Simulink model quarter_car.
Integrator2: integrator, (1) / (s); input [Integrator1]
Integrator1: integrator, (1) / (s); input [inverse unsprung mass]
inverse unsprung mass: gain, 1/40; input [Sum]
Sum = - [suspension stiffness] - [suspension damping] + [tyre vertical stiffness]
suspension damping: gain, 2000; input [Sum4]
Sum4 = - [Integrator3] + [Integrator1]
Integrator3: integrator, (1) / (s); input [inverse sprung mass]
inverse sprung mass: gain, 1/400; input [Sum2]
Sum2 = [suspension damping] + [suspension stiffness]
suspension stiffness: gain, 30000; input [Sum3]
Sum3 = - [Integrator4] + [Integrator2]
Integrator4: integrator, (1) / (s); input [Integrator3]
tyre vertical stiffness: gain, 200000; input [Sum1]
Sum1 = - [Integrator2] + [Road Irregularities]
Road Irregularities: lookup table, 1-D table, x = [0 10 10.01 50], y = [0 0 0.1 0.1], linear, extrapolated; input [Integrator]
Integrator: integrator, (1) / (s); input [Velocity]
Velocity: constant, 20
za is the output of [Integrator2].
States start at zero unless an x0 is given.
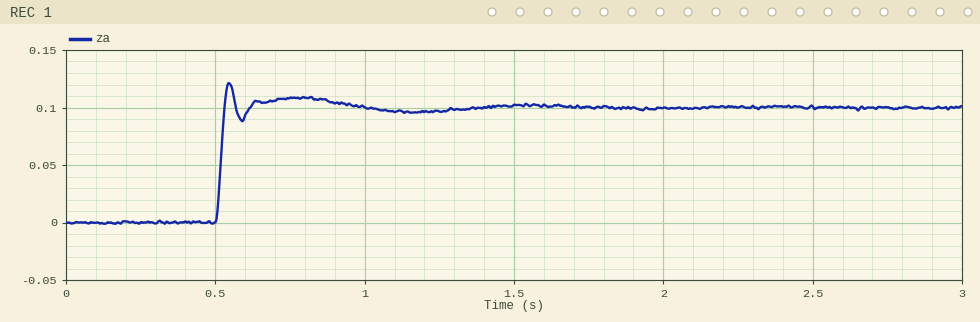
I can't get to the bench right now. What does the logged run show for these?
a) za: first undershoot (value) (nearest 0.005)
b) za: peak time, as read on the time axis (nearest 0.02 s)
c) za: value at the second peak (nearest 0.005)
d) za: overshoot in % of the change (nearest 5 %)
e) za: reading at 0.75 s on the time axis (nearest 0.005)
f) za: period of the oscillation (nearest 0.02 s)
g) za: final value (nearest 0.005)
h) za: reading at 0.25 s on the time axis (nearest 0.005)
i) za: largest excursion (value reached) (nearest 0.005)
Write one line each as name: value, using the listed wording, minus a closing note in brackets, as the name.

za: first undershoot (value): 0.090
za: peak time, as read on the time axis: 0.54 s
za: value at the second peak: 0.110
za: overshoot in % of the change: 20 %
za: reading at 0.75 s on the time axis: 0.110
za: period of the oscillation: 0.24 s
za: final value: 0.100
za: reading at 0.25 s on the time axis: 0.000
za: largest excursion (value reached): 0.120
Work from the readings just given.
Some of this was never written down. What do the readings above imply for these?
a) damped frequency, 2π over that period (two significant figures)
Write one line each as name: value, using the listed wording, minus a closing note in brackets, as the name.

damped frequency, 2π over that period: 26 rad/s
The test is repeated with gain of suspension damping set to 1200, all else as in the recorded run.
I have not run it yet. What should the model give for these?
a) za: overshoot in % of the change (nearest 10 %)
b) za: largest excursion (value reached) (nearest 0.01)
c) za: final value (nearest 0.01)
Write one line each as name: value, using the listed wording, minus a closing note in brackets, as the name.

za: overshoot in % of the change: 40 %
za: largest excursion (value reached): 0.14
za: final value: 0.10
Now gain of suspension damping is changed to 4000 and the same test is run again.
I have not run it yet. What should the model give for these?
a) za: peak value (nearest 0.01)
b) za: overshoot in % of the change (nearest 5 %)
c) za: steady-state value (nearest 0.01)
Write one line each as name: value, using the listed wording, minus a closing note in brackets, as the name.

za: peak value: 0.11
za: overshoot in % of the change: 10 %
za: steady-state value: 0.10
